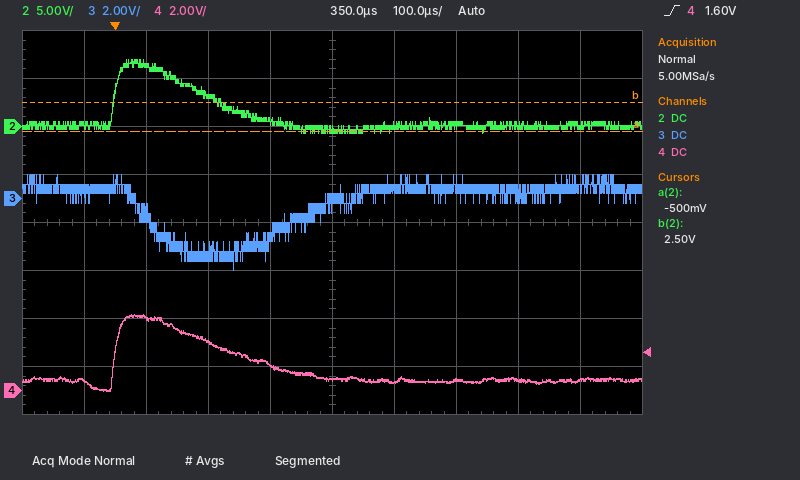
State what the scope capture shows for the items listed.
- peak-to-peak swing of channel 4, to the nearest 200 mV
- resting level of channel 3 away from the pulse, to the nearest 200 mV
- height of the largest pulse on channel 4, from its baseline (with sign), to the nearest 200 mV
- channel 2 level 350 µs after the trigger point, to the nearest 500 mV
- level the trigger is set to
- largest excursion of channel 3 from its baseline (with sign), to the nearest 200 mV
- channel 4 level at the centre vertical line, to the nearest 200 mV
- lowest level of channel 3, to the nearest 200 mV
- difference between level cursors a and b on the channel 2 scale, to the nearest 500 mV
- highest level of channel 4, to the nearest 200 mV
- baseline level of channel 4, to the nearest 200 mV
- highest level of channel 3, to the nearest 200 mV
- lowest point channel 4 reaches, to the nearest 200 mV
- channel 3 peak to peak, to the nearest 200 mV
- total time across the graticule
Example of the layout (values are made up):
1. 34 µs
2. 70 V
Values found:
1. 3.2 V
2. 400 mV
3. +2.8 V
4. -500 mV
5. 1.60 V
6. -3.4 V
7. 400 mV
8. -3.0 V
9. 3.0 V
10. 3.2 V
11. 400 mV
12. 1.0 V
13. 0.0 V
14. 4.0 V
15. 1 ms
